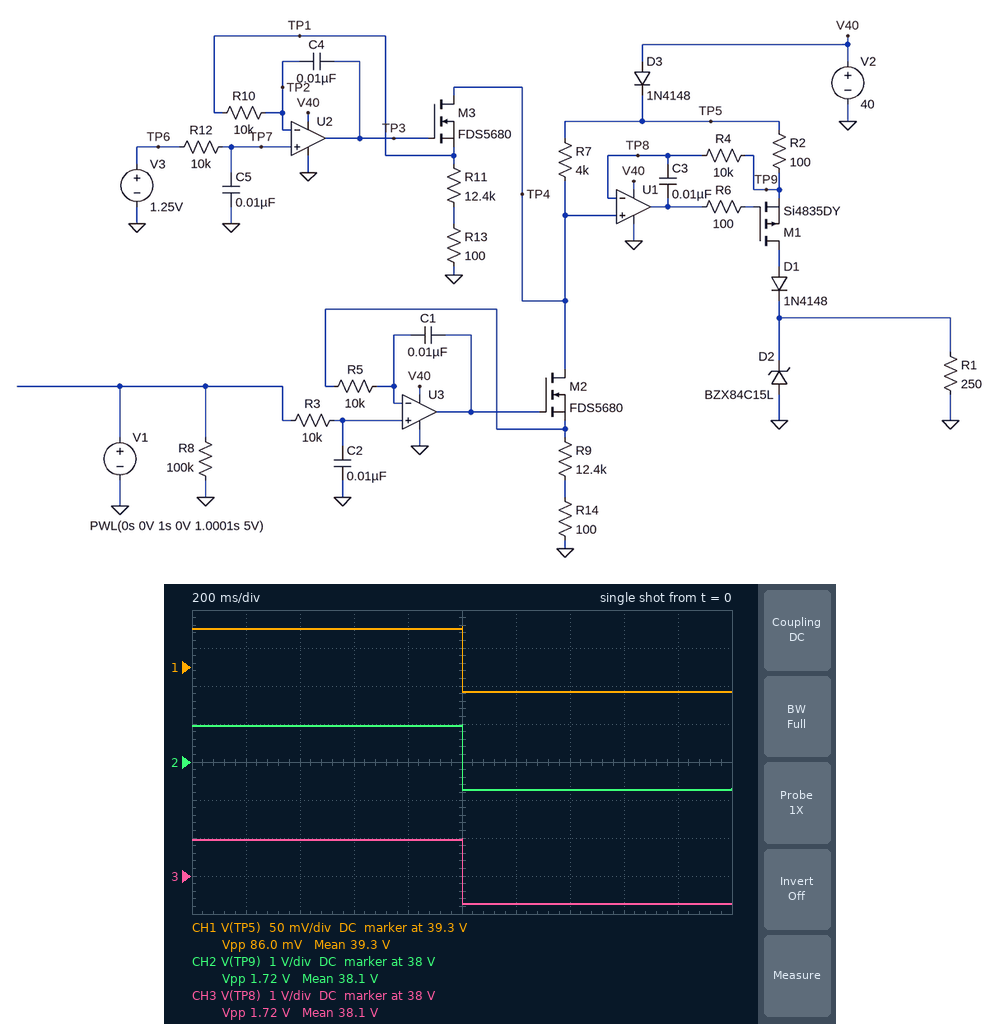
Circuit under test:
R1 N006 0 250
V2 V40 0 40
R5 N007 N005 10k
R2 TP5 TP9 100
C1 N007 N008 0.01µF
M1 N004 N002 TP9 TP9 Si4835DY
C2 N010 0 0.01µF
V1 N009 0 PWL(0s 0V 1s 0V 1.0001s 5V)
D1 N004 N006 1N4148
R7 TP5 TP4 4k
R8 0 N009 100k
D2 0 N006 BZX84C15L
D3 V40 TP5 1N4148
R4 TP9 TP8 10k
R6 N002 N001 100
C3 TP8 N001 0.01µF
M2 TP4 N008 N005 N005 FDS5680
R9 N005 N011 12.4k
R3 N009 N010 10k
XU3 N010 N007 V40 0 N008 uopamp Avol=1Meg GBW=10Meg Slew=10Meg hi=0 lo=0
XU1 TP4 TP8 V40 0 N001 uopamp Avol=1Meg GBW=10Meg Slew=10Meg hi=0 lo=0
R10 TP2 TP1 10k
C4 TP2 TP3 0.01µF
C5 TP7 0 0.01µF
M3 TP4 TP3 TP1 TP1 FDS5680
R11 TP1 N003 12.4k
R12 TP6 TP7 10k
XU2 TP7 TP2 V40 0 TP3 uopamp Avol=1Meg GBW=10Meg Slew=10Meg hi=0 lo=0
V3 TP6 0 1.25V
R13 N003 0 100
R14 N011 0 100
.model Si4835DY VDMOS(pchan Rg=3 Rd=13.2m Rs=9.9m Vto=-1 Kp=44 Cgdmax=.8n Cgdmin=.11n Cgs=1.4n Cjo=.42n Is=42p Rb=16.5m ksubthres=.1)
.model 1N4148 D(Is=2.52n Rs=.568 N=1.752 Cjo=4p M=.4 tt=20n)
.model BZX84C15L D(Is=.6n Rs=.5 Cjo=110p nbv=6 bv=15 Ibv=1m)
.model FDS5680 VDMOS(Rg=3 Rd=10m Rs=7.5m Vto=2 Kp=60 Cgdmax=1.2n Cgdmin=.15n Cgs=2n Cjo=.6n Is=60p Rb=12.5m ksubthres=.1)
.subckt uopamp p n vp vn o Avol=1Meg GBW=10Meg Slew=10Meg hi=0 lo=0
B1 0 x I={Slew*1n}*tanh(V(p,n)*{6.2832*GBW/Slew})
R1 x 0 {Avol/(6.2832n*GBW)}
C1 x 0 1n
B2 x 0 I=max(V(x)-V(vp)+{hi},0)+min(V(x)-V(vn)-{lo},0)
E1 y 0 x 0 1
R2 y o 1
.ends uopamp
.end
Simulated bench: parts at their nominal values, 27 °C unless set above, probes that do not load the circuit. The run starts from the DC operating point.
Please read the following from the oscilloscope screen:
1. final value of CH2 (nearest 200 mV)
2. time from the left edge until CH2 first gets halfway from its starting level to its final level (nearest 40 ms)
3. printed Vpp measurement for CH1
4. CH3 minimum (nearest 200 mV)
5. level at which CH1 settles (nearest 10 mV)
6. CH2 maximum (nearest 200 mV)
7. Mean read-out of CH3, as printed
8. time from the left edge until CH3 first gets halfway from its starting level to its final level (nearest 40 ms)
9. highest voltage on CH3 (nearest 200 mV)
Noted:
37.2 V
1.00 s
86.0 mV
37.2 V
39.27 V
39.0 V
38.1 V
1.00 s
39.0 V
